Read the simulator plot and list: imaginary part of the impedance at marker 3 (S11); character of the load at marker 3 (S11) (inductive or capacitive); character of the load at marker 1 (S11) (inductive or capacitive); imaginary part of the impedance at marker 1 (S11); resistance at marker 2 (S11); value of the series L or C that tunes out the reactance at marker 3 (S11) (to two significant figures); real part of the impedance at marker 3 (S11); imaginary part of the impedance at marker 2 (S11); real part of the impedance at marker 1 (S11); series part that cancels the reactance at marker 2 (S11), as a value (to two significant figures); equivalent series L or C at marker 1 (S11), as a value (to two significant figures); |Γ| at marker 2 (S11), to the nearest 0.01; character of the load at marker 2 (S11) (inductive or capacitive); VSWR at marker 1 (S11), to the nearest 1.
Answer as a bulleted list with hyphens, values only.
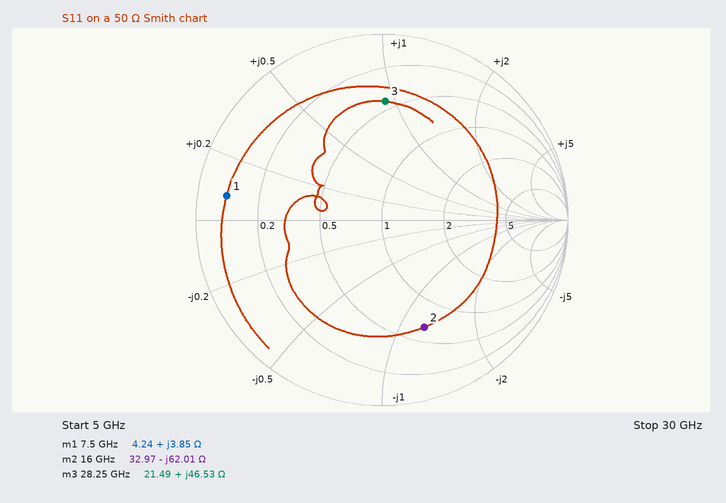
- +46.53 Ω
- inductive
- inductive
- +3.85 Ω
- 32.97 Ω
- 120 fF
- 21.49 Ω
- -62.01 Ω
- 4.24 Ω
- 620 pH
- 82 pH
- 0.62
- capacitive
- 12
